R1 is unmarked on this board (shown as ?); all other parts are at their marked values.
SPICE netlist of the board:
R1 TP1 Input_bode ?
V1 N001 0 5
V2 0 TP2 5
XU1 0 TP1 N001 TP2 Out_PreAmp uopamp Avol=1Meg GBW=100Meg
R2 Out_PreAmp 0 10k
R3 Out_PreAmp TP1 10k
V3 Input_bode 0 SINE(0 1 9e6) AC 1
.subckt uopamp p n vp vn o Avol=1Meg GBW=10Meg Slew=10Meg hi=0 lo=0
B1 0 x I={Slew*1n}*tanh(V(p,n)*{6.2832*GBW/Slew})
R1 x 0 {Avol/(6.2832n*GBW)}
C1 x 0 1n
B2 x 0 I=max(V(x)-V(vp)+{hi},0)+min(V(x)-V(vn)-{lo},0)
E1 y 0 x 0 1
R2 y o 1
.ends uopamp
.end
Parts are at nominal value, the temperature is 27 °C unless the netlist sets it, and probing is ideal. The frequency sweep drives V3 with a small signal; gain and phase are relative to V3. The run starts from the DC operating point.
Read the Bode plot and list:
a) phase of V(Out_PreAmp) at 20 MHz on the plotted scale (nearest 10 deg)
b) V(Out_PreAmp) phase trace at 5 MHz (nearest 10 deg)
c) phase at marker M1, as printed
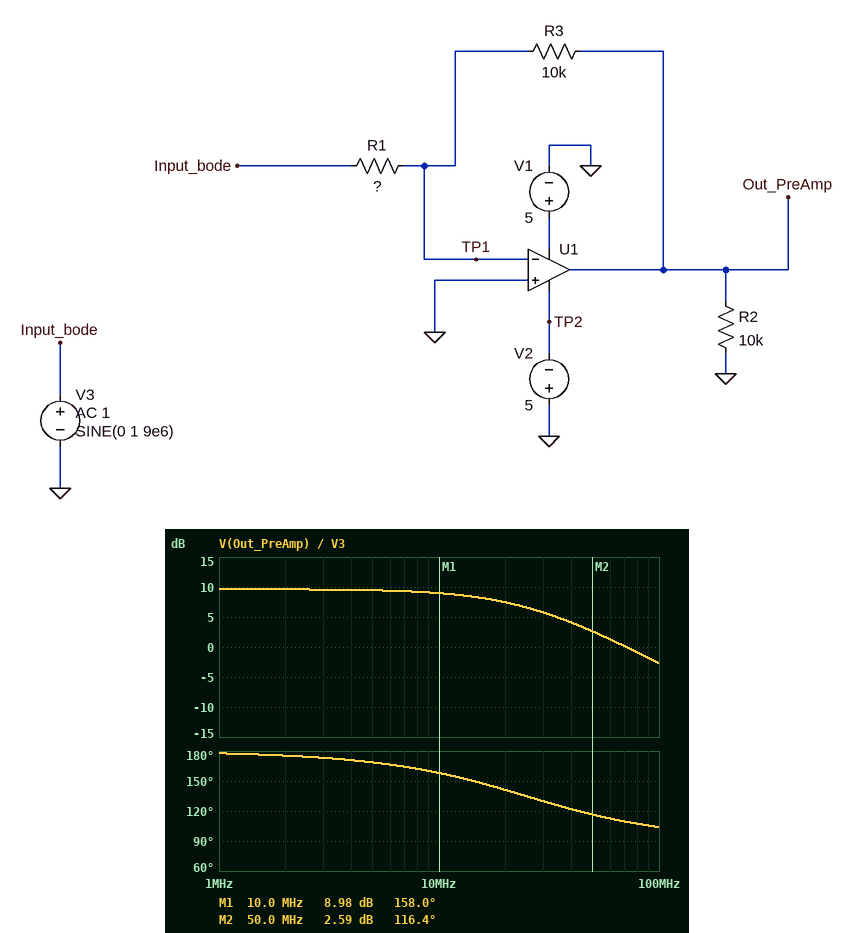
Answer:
140 deg
170 deg
158.0 deg
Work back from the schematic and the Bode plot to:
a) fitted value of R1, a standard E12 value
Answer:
3.3 kΩ
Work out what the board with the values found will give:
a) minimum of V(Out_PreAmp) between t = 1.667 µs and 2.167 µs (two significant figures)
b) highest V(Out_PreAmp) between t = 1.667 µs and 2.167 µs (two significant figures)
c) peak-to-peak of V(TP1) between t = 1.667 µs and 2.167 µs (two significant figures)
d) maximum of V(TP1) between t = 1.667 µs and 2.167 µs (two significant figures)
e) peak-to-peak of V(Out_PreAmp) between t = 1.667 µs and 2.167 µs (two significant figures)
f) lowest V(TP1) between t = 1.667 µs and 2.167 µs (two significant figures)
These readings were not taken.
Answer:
-280 mV
270 mV
1.5 V
750 mV
550 mV
-750 mV
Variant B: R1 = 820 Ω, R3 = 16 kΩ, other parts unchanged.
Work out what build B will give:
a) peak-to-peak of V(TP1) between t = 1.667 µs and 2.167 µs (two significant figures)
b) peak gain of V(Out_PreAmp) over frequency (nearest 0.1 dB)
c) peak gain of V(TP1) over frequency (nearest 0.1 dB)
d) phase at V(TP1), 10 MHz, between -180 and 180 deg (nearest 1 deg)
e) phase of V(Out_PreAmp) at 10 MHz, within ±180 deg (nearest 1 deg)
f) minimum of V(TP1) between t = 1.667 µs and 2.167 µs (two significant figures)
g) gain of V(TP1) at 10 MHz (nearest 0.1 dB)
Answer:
1.9 V
25.8 dB
-0.4 dB
26 deg
116 deg
-960 mV
-1.4 dB
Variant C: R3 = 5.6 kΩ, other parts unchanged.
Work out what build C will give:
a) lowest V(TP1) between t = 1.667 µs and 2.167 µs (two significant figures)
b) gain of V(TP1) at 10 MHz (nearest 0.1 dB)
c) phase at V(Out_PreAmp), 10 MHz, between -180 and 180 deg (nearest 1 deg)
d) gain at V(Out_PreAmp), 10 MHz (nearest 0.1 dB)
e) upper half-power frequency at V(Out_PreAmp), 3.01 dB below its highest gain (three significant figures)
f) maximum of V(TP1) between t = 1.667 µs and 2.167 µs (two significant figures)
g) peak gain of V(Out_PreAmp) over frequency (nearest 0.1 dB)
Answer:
-620 mV
-15.7 dB
165 deg
4.3 dB
37.1 MHz
620 mV
4.6 dB
